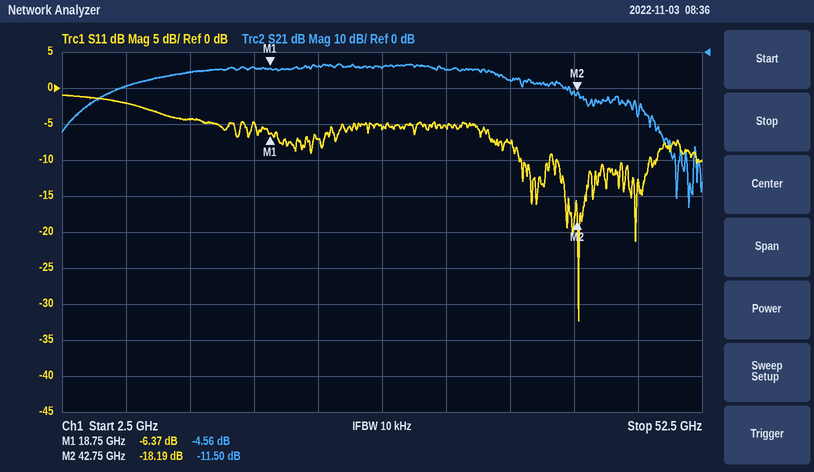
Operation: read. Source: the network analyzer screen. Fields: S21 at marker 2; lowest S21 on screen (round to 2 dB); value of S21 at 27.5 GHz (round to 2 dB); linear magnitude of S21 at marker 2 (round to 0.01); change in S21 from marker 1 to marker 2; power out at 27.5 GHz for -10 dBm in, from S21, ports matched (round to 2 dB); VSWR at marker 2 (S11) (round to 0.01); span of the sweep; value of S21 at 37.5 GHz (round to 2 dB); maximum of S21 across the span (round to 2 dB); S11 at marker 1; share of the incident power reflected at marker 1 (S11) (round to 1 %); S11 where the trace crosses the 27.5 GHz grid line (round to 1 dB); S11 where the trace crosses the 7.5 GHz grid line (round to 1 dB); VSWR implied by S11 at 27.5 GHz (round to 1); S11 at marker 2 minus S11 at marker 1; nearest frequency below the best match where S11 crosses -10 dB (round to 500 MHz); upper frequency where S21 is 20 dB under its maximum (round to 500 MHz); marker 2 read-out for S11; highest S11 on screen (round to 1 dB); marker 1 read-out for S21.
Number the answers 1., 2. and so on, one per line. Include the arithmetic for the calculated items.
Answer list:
1. -11.50 dB
2. -44 dB
3. -4 dB
4. 10^(-11.5/20) ≈ 0.27
5. -11.5 − (-4.56) = -6.94 dB
6. -10 dBm + (-4 dB) = -14 dBm
7. (1 + 0.1232)/(1 − 0.1232) ≈ 1.28
8. 50 GHz
9. -8 dB
10. -4 dB
11. -6.37 dB
12. 10^(-6.37/10) ≈ 23 %
13. -6 dB
14. -2 dB
15. |Γ| = 10^(-6/20) = 0.5012; VSWR = (1 + 0.5012)/(1 − 0.5012) ≈ 3
16. -18.19 − (-6.37) = -11.82 dB
17. 41.0 GHz
18. 49.5 GHz
19. -18.19 dB
20. -1 dB
21. -4.56 dB
